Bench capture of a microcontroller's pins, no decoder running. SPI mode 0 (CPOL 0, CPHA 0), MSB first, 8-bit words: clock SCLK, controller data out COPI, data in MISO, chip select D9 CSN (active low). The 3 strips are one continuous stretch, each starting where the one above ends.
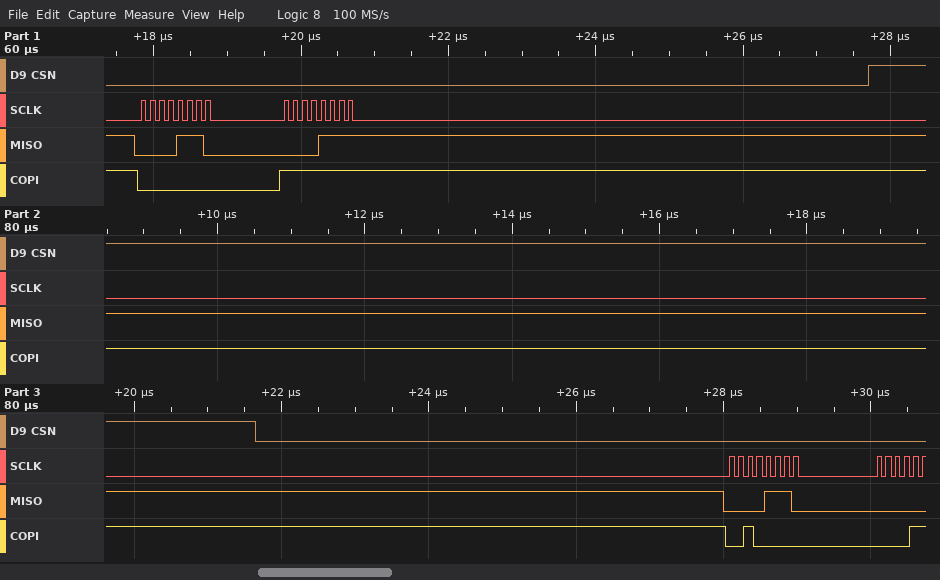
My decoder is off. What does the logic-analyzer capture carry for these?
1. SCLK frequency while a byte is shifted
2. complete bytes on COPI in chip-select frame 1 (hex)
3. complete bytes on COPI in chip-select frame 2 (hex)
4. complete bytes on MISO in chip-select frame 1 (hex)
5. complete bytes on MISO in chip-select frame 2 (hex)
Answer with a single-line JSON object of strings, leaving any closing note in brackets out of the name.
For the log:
{"SCLK frequency while a byte is shifted": "8 MHz", "complete bytes on COPI in chip-select frame 1": "00 FF", "complete bytes on COPI in chip-select frame 2": "20", "complete bytes on MISO in chip-select frame 1": "0E 0F", "complete bytes on MISO in chip-select frame 2": "0E"}
